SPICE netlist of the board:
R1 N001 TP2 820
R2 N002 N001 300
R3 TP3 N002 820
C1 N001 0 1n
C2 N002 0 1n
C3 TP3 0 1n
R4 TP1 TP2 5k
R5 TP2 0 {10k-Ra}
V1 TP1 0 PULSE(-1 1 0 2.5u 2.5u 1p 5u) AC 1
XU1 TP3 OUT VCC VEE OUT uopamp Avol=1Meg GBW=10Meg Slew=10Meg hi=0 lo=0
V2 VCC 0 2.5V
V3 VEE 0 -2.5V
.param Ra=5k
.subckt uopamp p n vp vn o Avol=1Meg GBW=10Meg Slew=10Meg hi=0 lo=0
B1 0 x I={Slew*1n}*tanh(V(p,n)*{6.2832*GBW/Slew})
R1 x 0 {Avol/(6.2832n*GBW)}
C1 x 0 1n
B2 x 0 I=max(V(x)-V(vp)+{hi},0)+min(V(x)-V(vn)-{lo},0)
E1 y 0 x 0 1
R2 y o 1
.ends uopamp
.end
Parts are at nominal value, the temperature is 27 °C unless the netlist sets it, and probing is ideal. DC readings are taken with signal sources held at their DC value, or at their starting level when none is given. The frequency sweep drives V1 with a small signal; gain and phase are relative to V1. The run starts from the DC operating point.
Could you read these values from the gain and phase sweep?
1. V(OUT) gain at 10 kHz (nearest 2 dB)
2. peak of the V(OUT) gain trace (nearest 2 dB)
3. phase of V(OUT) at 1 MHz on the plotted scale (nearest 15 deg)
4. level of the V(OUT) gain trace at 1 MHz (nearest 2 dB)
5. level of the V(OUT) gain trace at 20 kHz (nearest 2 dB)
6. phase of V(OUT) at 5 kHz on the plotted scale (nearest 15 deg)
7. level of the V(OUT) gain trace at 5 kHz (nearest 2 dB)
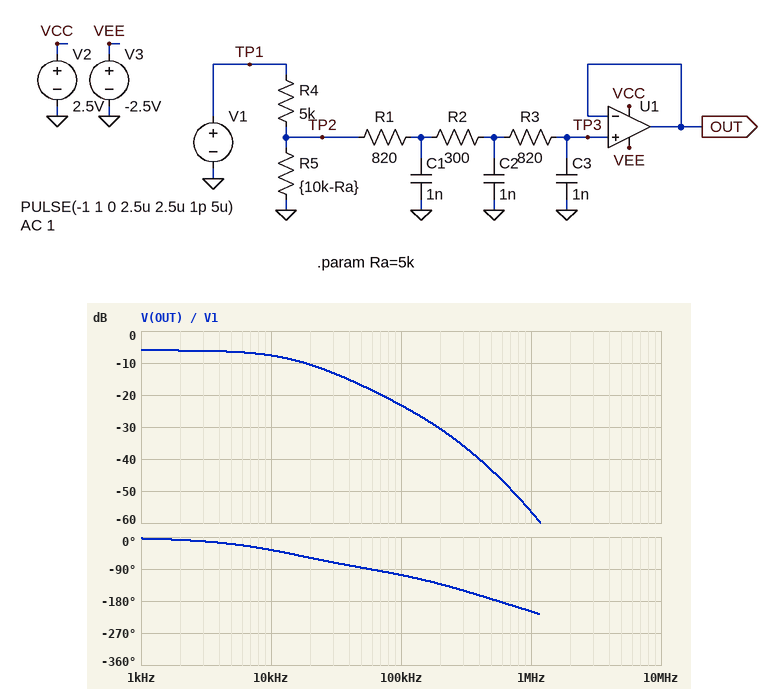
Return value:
-8 dB
-6 dB
-210 deg
-56 dB
-10 dB
-15 deg
-6 dB
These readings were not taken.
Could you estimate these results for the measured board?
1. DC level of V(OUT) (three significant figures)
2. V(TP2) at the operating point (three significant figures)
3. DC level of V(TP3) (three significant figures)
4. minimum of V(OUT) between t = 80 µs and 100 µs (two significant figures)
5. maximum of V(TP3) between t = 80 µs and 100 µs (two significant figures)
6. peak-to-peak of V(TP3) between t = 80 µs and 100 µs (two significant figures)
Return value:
-500 mV
-500 mV
-500 mV
-24 mV
24 mV
48 mV
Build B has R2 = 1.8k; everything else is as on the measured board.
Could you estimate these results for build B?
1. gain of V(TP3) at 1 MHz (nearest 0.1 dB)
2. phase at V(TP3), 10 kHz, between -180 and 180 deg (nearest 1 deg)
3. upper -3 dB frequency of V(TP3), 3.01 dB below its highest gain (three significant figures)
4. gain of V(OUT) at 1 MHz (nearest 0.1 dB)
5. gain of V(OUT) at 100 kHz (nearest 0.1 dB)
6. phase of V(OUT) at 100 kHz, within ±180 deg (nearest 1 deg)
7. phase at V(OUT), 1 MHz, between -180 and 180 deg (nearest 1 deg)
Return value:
-68.6 dB
-44 deg
12.2 kHz
-68.7 dB
-26.1 dB
-130 deg
118 deg
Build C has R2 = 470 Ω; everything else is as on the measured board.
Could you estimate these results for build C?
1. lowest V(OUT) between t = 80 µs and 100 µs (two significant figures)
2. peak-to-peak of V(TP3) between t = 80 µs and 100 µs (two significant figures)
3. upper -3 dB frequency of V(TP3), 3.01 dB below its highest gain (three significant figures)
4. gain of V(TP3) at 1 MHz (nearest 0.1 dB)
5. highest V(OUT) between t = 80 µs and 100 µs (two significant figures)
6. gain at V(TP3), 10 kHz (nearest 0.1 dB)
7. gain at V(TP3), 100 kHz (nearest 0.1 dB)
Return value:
-23 mV
45 mV
14.5 kHz
-58.7 dB
22 mV
-7.7 dB
-23.5 dB
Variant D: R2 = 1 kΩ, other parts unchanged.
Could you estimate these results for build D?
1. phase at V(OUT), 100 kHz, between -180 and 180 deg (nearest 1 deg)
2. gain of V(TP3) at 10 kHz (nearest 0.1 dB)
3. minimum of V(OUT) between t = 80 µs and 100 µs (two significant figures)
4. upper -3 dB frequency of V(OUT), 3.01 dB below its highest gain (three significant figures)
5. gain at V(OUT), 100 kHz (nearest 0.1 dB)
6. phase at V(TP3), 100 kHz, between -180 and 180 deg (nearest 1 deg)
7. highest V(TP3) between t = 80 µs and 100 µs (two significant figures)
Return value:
-120 deg
-7.9 dB
-19 mV
13.5 kHz
-24.5 dB
-119 deg
18 mV
